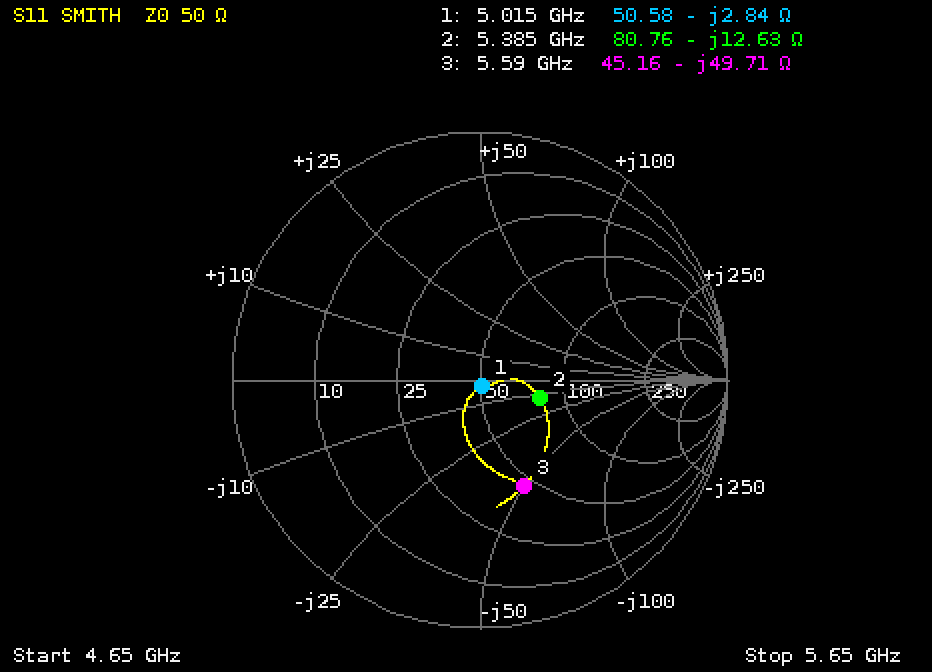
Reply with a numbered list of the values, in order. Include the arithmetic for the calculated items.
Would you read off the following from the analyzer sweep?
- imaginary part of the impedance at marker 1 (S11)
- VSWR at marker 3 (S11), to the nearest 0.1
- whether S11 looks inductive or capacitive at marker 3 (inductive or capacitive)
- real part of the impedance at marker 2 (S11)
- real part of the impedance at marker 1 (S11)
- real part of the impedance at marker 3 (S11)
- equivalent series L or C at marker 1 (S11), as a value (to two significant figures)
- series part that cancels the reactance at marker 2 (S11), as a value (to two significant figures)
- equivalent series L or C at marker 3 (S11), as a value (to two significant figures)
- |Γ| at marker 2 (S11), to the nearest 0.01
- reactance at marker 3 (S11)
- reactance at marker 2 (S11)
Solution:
1. -2.84 Ω
2. 2.7
3. capacitive
4. 80.76 Ω
5. 50.58 Ω
6. 45.16 Ω
7. C = 1/(2π × 5.015 GHz × 2.84 Ω) ≈ 11 pF
8. L = 12.63 Ω/(2π × 5.385 GHz) ≈ 373 pH, so 370 pH to two significant figures
9. C = 1/(2π × 5.59 GHz × 49.71 Ω) ≈ 573 fF, so 570 fF to two significant figures
10. 0.25
11. -49.71 Ω
12. -12.63 Ω
